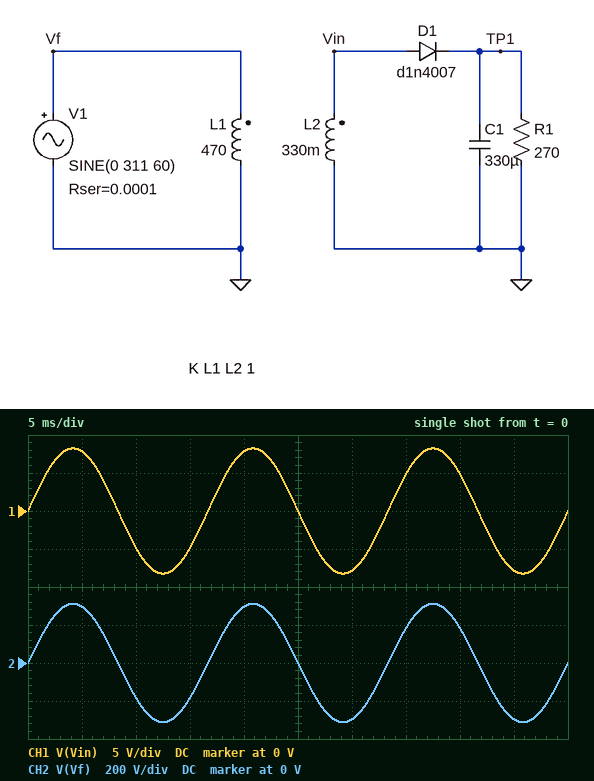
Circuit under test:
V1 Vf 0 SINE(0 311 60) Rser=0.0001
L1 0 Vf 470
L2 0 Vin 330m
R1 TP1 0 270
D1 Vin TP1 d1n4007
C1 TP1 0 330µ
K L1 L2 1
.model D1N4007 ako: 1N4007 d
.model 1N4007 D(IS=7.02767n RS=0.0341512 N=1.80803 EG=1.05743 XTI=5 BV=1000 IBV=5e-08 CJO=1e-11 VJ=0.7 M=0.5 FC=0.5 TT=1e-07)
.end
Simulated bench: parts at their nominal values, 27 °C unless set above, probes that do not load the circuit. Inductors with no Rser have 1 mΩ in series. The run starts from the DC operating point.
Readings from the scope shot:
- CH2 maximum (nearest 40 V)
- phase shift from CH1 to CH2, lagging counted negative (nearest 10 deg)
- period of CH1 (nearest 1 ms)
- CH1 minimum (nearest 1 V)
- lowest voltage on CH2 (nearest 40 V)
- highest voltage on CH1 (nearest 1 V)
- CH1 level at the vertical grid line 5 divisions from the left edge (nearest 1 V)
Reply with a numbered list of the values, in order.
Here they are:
1. 320 V
2. 0 deg
3. 17 ms
4. -8 V
5. -320 V
6. 8 V
7. 0 V
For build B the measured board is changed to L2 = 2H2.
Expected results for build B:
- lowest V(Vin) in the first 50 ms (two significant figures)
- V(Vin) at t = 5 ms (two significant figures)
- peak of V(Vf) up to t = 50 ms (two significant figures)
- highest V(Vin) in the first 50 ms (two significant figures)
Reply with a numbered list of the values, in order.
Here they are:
1. -21 V
2. 20 V
3. 310 V
4. 21 V
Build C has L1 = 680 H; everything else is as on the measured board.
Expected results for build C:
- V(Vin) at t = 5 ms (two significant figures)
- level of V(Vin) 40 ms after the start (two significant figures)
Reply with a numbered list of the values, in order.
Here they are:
1. 6.5 V
2. 4.0 V
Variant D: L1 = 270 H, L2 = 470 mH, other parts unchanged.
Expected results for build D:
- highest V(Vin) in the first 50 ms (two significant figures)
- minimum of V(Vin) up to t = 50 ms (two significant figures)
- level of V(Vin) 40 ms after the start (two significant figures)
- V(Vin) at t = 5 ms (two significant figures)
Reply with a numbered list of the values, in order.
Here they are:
1. 13 V
2. -13 V
3. 7.6 V
4. 12 V
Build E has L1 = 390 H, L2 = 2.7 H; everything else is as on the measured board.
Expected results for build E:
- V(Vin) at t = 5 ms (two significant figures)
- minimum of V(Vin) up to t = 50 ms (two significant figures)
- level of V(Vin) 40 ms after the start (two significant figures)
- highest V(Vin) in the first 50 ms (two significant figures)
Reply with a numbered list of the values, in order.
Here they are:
1. 25 V
2. -26 V
3. 15 V
4. 26 V
